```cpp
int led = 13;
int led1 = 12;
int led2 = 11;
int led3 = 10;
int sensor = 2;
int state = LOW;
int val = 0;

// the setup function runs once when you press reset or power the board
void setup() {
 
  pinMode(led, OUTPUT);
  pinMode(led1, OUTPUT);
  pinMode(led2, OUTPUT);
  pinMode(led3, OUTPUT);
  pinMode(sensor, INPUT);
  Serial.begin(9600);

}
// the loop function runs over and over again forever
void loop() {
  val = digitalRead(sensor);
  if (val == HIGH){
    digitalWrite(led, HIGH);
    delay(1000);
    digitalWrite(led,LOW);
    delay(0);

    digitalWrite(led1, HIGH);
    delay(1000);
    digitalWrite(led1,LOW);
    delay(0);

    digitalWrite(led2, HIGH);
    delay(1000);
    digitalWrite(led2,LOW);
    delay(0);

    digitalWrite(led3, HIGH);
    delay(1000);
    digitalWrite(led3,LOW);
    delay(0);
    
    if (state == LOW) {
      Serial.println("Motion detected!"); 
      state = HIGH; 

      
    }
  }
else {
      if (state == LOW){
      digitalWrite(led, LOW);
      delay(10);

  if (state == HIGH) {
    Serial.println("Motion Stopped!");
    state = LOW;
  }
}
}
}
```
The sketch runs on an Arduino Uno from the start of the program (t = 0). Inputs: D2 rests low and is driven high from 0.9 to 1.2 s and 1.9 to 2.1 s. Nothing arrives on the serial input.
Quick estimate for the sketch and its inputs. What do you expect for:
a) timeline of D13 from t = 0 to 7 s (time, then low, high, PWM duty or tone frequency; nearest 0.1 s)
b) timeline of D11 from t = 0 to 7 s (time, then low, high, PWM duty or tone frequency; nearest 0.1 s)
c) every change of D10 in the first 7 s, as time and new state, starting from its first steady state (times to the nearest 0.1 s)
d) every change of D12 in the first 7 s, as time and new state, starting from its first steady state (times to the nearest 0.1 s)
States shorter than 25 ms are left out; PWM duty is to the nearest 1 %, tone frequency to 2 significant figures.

0 s low; 0.9 s high; 1.9 s low
0 s low; 2.9 s high; 3.9 s low
0 s low; 3.9 s high; 4.9 s low
0 s low; 1.9 s high; 2.9 s low
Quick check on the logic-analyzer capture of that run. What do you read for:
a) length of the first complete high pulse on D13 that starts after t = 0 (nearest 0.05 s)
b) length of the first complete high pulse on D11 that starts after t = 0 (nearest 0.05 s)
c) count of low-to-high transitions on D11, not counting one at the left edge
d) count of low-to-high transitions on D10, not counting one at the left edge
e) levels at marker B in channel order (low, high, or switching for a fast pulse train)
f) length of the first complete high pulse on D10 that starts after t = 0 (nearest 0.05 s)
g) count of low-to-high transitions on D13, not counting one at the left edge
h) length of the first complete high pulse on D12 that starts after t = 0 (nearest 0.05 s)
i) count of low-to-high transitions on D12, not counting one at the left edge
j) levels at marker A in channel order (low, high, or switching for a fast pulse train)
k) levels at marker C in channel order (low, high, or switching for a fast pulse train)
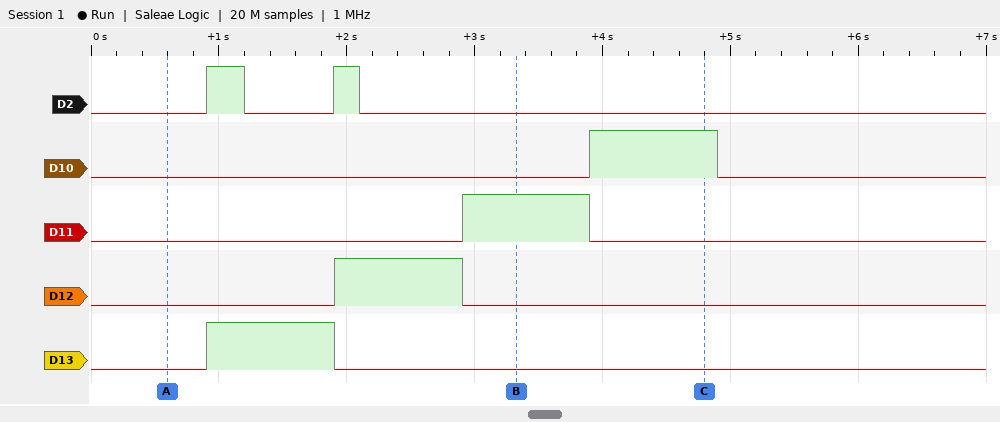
1.00 s
1.00 s
1
1
D2 low, D10 low, D11 high, D12 low, D13 low
1.00 s
1
1.00 s
1
D2 low, D10 low, D11 low, D12 low, D13 low
D2 low, D10 high, D11 low, D12 low, D13 low
